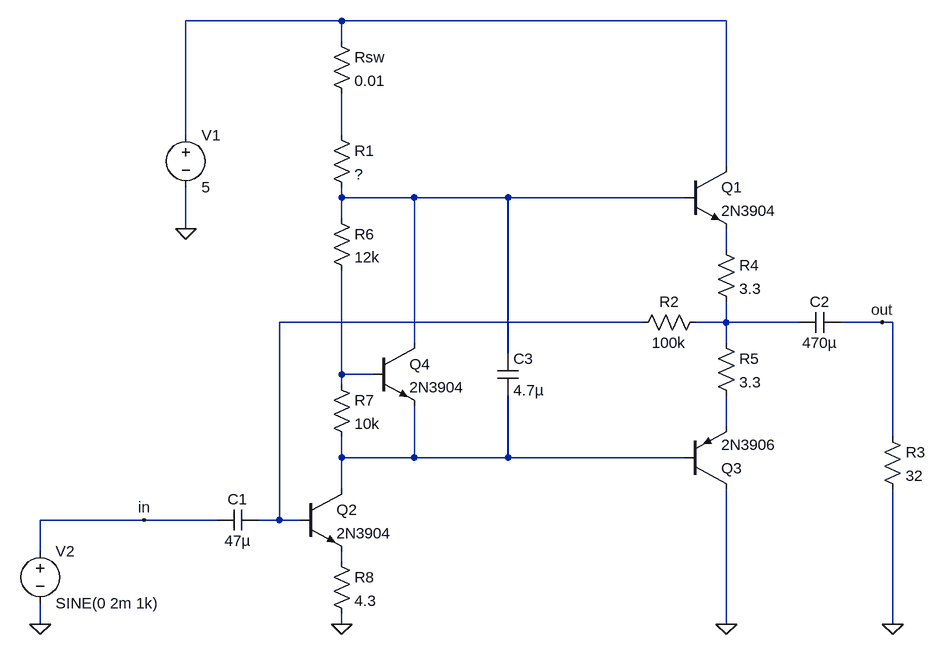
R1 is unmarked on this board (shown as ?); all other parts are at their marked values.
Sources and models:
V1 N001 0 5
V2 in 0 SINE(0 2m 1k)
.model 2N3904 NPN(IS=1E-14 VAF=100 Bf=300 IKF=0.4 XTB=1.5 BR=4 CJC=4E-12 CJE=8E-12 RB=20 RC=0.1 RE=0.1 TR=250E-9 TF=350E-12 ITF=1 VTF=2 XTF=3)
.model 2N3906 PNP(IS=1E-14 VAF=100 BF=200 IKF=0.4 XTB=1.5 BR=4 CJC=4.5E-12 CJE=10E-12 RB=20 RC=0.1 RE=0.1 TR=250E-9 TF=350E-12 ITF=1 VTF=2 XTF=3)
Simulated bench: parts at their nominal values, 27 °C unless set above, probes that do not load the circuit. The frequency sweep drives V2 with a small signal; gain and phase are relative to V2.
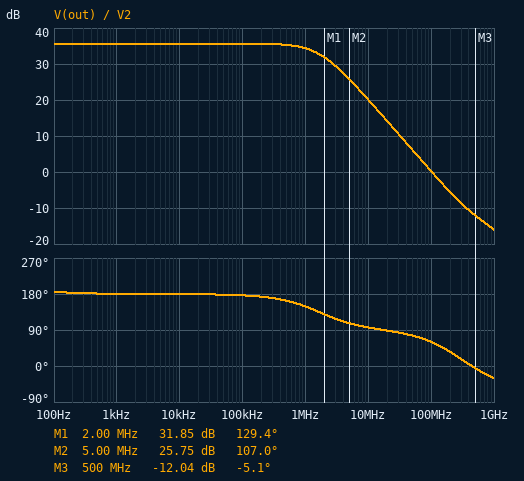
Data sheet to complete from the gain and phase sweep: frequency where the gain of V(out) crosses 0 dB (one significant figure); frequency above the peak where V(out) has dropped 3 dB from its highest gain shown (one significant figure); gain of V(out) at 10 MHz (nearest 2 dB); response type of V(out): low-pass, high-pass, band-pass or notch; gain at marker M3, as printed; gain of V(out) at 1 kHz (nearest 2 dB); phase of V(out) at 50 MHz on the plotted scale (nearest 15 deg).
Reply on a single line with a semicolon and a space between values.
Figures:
100 MHz; 2 MHz; 20 dB; low-pass; -12.04 dB; 36 dB; 75 deg
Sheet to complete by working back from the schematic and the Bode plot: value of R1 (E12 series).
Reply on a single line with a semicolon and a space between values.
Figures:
4.7 kΩ
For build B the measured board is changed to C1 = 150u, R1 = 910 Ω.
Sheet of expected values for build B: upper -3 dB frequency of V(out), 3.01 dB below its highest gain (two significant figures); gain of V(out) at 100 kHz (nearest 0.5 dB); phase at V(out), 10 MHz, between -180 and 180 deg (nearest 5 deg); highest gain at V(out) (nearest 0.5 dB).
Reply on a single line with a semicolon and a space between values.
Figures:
7.3 MHz; 34.5 dB; 125 deg; 35.0 dB
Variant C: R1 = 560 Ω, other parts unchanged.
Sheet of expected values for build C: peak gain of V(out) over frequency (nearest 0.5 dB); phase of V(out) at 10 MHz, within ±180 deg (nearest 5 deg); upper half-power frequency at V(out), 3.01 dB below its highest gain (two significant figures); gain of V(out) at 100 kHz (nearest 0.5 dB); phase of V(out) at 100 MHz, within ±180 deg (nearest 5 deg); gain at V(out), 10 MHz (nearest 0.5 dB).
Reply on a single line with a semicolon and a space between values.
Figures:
33.0 dB; 135 deg; 11 MHz; 32.5 dB; 75 deg; 30.0 dB
